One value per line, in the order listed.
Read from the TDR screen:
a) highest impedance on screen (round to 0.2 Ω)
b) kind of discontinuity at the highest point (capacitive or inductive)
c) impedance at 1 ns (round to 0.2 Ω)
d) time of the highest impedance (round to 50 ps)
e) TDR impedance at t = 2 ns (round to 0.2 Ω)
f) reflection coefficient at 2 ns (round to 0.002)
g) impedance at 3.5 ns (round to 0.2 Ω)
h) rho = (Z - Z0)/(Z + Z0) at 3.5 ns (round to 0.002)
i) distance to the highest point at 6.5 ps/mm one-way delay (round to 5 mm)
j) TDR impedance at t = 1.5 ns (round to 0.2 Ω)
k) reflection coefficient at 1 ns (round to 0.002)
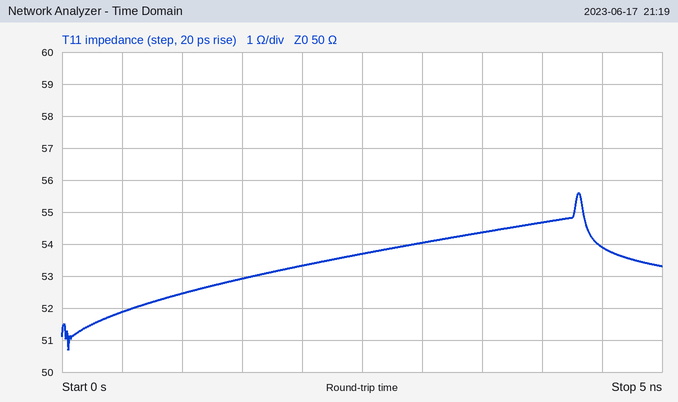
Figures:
55.6 Ω
inductive
52.4 Ω
4.30 ns
53.4 Ω
+0.032
54.4 Ω
+0.042
330 mm
53.0 Ω
+0.024
